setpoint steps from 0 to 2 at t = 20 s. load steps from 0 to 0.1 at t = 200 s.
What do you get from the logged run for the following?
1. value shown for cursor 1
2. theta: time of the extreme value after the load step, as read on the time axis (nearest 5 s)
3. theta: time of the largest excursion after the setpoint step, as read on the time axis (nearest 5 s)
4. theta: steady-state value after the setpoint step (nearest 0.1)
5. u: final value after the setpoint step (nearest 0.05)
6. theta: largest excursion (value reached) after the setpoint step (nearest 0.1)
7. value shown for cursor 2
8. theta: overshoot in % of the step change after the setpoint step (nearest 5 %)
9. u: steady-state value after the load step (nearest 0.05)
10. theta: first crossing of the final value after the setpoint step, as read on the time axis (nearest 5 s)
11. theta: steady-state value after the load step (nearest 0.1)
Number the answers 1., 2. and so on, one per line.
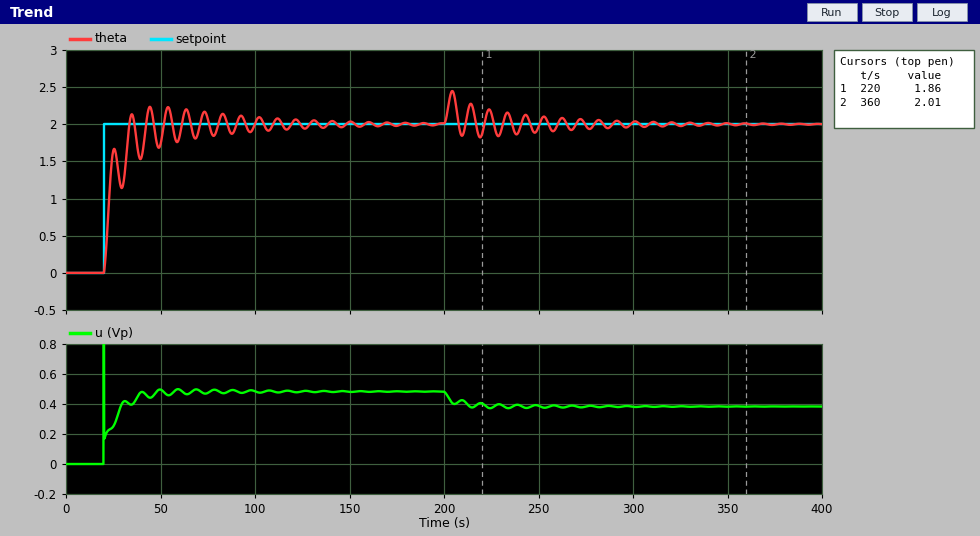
1. 1.86
2. 205 s
3. 45 s
4. 2.0
5. 0.50
6. 2.2
7. 2.01
8. 10 %
9. 0.40
10. 35 s
11. 2.0
